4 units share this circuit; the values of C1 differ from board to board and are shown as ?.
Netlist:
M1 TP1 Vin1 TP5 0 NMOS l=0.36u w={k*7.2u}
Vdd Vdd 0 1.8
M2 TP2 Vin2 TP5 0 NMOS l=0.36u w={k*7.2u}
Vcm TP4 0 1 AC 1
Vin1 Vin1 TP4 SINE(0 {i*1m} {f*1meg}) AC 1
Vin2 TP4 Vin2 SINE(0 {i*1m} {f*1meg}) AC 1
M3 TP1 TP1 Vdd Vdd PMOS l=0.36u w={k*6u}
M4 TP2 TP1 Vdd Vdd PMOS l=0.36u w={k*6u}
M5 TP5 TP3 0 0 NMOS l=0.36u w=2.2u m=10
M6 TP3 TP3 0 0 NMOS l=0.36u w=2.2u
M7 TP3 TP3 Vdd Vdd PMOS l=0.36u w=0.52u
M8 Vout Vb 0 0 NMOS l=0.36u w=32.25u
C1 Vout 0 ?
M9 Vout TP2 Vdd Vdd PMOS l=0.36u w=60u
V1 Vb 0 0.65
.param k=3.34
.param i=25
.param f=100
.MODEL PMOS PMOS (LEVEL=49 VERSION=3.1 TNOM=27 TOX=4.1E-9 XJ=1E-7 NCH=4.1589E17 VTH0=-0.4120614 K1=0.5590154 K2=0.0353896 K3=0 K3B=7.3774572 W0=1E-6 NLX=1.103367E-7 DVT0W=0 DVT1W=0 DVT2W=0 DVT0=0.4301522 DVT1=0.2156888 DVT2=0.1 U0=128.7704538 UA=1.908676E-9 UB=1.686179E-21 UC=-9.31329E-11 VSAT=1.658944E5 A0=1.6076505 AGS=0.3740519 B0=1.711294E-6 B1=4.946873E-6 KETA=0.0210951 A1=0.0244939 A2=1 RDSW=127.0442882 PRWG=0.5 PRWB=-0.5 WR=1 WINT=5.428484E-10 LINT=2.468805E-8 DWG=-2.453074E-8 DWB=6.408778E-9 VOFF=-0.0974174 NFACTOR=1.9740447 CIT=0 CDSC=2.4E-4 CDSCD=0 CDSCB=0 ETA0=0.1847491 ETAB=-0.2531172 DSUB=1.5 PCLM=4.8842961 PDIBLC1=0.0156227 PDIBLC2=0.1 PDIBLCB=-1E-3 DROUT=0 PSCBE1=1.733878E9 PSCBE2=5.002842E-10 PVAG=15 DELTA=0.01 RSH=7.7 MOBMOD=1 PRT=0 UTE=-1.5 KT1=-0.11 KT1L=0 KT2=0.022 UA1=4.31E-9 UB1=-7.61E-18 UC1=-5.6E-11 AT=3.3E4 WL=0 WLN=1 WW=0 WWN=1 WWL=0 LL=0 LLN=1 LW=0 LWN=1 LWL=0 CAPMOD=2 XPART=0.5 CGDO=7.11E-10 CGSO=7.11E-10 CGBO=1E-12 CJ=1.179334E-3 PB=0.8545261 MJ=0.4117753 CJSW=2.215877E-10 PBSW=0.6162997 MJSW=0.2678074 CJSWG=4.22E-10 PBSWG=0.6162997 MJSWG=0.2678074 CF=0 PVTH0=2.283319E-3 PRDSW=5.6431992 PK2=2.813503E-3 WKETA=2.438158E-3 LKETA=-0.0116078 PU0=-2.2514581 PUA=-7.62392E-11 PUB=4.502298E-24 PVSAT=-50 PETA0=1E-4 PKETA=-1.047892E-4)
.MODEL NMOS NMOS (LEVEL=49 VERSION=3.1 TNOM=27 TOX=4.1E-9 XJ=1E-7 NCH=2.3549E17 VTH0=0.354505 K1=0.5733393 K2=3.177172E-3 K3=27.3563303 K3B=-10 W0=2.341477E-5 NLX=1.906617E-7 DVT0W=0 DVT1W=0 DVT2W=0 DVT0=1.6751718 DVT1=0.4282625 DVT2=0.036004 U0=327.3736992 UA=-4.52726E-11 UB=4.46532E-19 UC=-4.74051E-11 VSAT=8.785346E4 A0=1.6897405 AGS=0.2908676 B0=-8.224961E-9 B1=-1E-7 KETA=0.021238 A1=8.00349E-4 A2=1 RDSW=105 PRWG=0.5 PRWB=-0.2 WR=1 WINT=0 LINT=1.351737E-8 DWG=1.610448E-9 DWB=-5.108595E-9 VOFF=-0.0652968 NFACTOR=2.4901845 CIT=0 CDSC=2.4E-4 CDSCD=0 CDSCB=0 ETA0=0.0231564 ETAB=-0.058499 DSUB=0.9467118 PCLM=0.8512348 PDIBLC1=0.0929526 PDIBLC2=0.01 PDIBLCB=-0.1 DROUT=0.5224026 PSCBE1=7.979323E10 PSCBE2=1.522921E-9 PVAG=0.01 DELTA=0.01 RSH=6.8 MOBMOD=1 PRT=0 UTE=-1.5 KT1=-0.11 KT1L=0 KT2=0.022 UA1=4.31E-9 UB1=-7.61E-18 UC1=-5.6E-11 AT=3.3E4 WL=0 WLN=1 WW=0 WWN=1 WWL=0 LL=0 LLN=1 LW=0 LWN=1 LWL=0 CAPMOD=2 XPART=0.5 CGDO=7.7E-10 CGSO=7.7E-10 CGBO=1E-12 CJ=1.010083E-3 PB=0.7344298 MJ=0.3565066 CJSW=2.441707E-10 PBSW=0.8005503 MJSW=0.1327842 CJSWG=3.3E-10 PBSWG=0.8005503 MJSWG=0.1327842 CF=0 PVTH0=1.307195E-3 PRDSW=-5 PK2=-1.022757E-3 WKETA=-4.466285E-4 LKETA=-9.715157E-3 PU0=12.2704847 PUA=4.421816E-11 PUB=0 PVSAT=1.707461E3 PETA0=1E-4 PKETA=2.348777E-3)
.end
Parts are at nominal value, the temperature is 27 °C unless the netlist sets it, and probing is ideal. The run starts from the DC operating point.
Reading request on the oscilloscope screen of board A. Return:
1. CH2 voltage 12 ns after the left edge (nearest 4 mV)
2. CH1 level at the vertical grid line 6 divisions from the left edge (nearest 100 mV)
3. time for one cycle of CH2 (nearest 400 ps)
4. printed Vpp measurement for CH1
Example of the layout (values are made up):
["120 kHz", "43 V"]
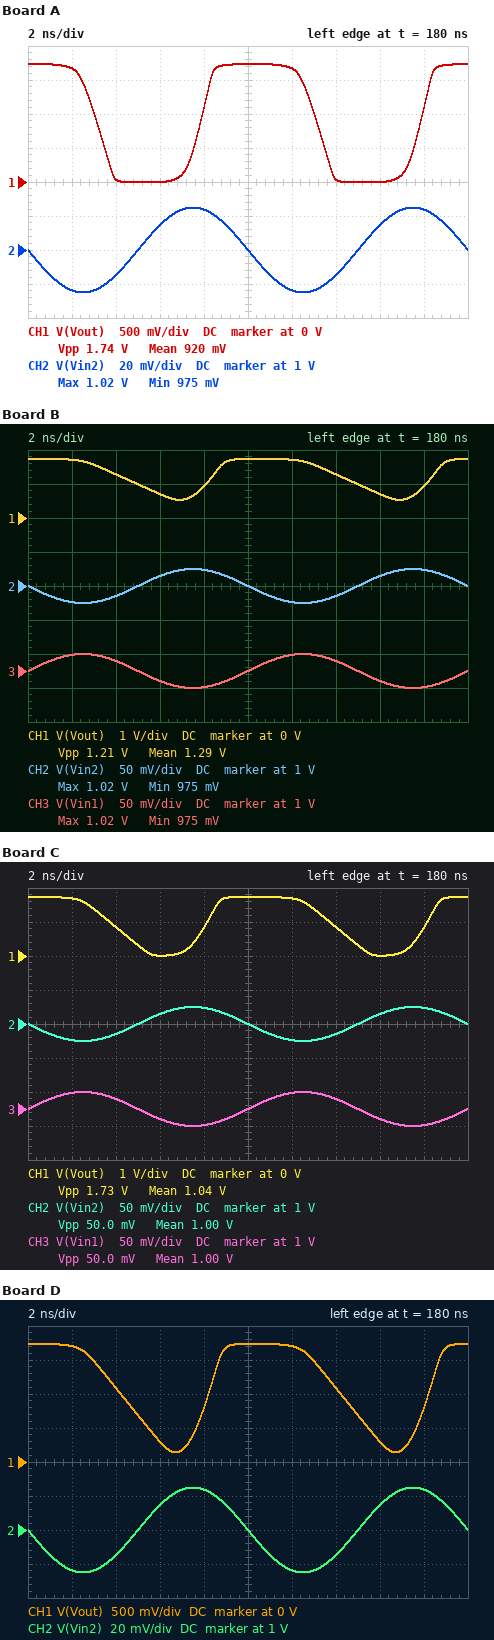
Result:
["976 mV", "1.7 V", "10.0 ns", "1.74 V"]
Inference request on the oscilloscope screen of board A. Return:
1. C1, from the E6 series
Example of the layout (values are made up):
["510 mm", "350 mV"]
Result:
["150 fF"]
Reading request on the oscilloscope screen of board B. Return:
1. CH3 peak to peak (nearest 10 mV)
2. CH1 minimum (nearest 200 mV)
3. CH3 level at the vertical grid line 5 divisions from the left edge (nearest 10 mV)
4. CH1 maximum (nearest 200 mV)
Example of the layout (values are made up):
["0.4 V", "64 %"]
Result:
["50 mV", "600 mV", "1.00 V", "1.8 V"]
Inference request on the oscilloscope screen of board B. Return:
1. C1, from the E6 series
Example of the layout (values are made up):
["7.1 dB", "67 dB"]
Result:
["1 pF"]
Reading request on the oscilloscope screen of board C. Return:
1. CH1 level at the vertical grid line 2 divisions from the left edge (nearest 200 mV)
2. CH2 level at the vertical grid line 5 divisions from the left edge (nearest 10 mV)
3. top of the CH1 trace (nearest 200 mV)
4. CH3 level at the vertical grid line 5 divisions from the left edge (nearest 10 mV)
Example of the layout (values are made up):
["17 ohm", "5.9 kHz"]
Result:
["800 mV", "1.00 V", "1.8 V", "1.00 V"]
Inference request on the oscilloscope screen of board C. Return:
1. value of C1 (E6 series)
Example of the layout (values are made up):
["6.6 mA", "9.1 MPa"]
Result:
["470 fF"]
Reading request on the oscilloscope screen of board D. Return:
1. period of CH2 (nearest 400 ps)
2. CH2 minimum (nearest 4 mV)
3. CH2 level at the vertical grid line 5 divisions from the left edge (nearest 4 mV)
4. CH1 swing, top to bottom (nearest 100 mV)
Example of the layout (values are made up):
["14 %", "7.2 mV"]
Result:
["10.0 ns", "976 mV", "1.000 V", "1.6 V"]
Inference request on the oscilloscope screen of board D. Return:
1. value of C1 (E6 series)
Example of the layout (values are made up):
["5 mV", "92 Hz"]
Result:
["680 fF"]
